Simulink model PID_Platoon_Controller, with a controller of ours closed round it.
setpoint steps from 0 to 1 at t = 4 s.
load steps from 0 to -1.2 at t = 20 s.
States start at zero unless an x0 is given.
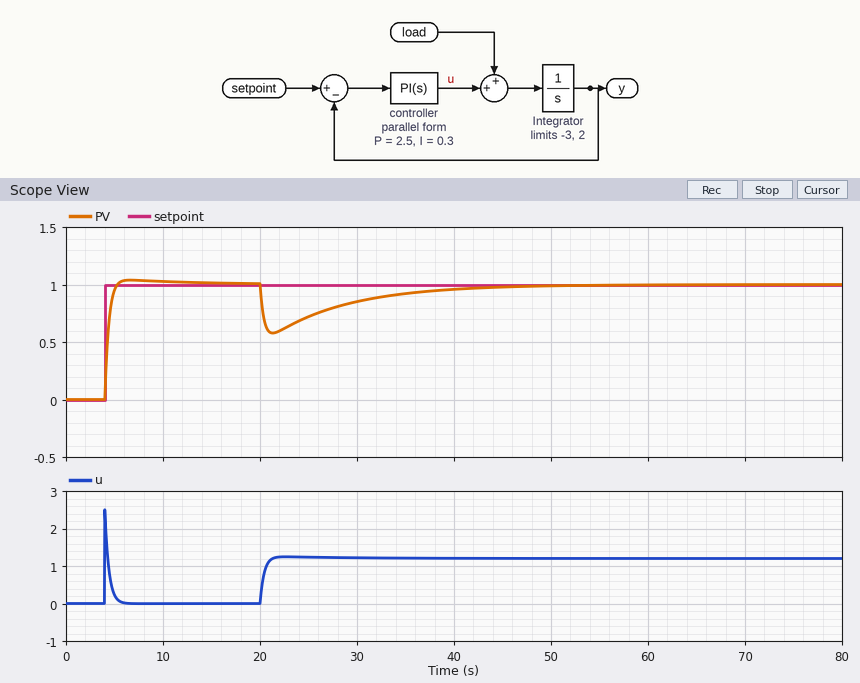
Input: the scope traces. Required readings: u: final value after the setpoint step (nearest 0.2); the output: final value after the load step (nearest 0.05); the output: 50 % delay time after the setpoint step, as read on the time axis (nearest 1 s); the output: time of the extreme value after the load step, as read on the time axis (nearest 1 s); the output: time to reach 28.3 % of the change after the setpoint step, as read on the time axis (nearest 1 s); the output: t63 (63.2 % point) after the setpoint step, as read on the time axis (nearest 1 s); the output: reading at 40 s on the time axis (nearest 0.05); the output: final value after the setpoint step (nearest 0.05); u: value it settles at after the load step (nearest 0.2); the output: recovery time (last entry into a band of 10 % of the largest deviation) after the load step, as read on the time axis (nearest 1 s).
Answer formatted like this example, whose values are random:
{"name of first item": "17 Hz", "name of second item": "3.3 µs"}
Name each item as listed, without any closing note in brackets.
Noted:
{"u: final value after the setpoint step": "0.0", "the output: final value after the load step": "1.00", "the output: 50 % delay time after the setpoint step, as read on the time axis": "4 s", "the output: time of the extreme value after the load step, as read on the time axis": "21 s", "the output: time to reach 28.3 % of the change after the setpoint step, as read on the time axis": "4 s", "the output: t63 (63.2 % point) after the setpoint step, as read on the time axis": "4 s", "the output: reading at 40 s on the time axis": "0.95", "the output: final value after the setpoint step": "1.00", "u: value it settles at after the load step": "1.2", "the output: recovery time (last entry into a band of 10 % of the largest deviation) after the load step, as read on the time axis": "40 s"}
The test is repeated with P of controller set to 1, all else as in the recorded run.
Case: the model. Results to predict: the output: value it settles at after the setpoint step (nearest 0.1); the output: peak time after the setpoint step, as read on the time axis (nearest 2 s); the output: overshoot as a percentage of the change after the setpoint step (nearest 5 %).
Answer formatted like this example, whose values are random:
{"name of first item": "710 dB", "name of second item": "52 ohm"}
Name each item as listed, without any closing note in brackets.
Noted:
{"the output: value it settles at after the setpoint step": "1.0", "the output: peak time after the setpoint step, as read on the time axis": "8 s", "the output: overshoot as a percentage of the change after the setpoint step": "15 %"}
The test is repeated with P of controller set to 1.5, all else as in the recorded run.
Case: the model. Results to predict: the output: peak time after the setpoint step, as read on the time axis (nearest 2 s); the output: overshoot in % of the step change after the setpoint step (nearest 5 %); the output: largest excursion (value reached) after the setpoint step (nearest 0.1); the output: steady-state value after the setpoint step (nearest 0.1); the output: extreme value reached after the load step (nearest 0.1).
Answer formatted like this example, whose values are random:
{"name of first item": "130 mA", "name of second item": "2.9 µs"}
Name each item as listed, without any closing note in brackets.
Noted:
{"the output: peak time after the setpoint step, as read on the time axis": "8 s", "the output: overshoot in % of the step change after the setpoint step": "10 %", "the output: largest excursion (value reached) after the setpoint step": "1.1", "the output: steady-state value after the setpoint step": "1.0", "the output: extreme value reached after the load step": "0.4"}
